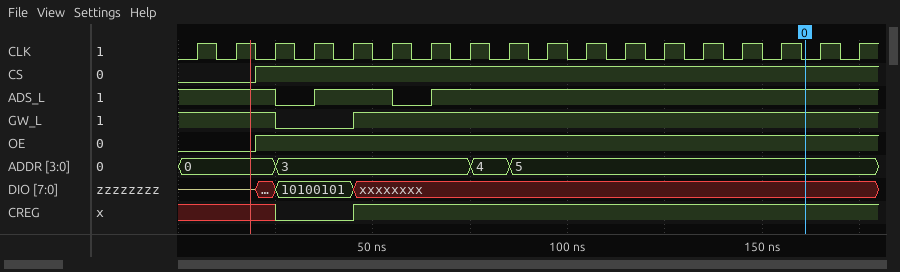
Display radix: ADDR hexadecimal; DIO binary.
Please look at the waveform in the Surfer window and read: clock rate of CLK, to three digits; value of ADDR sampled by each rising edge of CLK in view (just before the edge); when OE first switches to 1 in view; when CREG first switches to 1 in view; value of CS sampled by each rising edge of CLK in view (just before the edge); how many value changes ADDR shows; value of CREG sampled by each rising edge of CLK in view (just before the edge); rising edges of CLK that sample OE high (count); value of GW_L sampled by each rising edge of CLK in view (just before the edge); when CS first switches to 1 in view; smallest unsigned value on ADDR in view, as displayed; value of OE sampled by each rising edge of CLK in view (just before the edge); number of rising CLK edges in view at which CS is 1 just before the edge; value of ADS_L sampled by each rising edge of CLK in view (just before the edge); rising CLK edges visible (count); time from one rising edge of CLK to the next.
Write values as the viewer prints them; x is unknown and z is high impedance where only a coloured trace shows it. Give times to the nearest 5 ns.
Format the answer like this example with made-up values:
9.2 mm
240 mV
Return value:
100 MHz
0, 0, 0, 3, 3, 3, 3, 3, 4, 5, 5, 5, 5, 5, 5, 5, 5, 5
20 ns
45 ns
0 0 1 1 1 1 1 1 1 1 1 1 1 1 1 1 1 1
3
x x x 0 0 1 1 1 1 1 1 1 1 1 1 1 1 1
16
1 1 1 0 0 1 1 1 1 1 1 1 1 1 1 1 1 1
20 ns
0
0 0 1 1 1 1 1 1 1 1 1 1 1 1 1 1 1 1
16
1 1 1 0 1 1 0 1 1 1 1 1 1 1 1 1 1 1
18
10 ns
